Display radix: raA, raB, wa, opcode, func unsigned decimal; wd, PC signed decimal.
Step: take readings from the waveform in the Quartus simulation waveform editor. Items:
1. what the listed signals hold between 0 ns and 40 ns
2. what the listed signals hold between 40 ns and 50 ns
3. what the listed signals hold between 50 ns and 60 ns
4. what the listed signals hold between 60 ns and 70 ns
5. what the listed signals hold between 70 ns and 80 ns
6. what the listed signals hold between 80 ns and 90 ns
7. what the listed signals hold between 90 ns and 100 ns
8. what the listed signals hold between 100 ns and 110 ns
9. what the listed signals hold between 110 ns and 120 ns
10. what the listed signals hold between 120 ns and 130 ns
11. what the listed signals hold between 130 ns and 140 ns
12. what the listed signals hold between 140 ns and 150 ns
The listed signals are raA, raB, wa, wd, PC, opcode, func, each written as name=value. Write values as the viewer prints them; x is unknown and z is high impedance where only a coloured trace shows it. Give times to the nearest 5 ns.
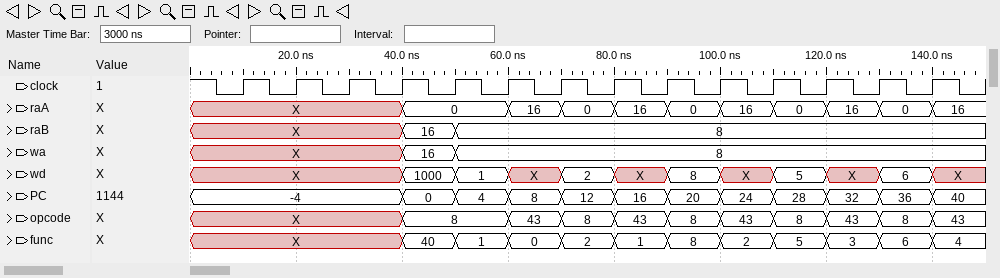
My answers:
raA=X, raB=X, wa=X, wd=X, PC=-4, opcode=X, func=X
raA=0, raB=16, wa=16, wd=1000, PC=0, opcode=8, func=40
raA=0, raB=8, wa=8, wd=1, PC=4, opcode=8, func=1
raA=16, raB=8, wa=8, wd=X, PC=8, opcode=43, func=0
raA=0, raB=8, wa=8, wd=2, PC=12, opcode=8, func=2
raA=16, raB=8, wa=8, wd=X, PC=16, opcode=43, func=1
raA=0, raB=8, wa=8, wd=8, PC=20, opcode=8, func=8
raA=16, raB=8, wa=8, wd=X, PC=24, opcode=43, func=2
raA=0, raB=8, wa=8, wd=5, PC=28, opcode=8, func=5
raA=16, raB=8, wa=8, wd=X, PC=32, opcode=43, func=3
raA=0, raB=8, wa=8, wd=6, PC=36, opcode=8, func=6
raA=16, raB=8, wa=8, wd=X, PC=40, opcode=43, func=4
